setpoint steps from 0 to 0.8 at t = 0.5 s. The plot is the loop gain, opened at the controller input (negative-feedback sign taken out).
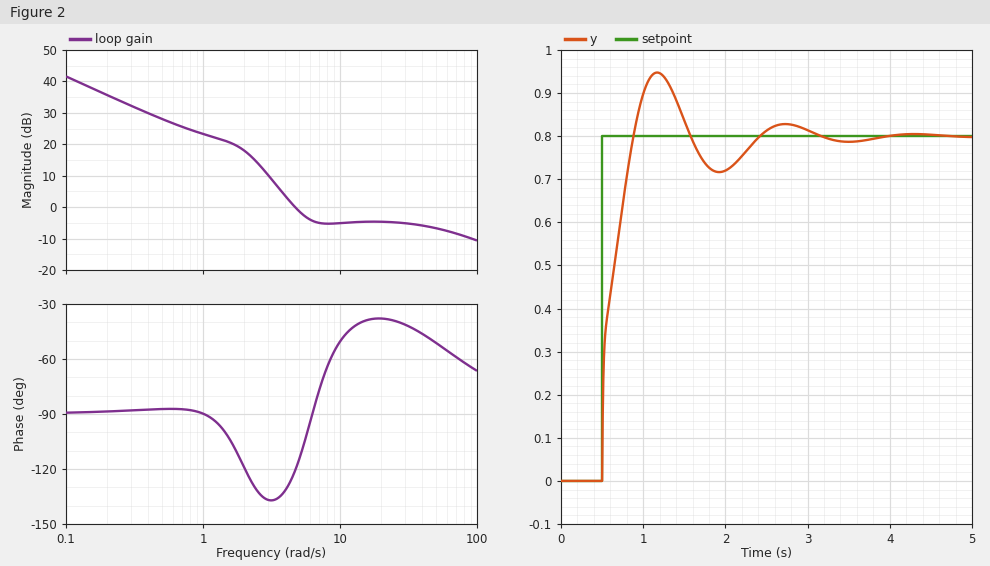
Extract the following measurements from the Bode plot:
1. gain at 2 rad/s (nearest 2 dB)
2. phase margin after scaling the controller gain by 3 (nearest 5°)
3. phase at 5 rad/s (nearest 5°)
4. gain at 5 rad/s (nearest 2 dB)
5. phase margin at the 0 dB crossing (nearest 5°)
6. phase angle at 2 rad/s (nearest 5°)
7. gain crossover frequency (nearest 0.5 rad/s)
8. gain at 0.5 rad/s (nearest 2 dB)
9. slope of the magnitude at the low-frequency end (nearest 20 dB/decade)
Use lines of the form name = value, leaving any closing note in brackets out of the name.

gain at 2 rad/s = 18 dB
phase margin after scaling the controller gain by 3 = 115°
phase at 5 rad/s = -115°
gain at 5 rad/s = -2 dB
phase margin at the 0 dB crossing = 60°
phase angle at 2 rad/s = -120°
gain crossover frequency = 4.5 rad/s
gain at 0.5 rad/s = 28 dB
slope of the magnitude at the low-frequency end = -20 dB/decade
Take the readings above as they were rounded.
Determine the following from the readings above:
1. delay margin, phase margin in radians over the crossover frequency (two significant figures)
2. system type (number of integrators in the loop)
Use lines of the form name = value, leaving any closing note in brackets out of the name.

delay margin, phase margin in radians over the crossover frequency = 0.23 s
system type = 1
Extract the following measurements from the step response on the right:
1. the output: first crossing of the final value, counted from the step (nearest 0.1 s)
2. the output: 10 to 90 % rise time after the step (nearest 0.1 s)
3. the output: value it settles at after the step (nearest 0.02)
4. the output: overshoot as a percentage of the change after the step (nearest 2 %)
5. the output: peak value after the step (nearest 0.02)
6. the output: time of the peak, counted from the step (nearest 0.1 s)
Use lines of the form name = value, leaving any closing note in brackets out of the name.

the output: first crossing of the final value, counted from the step = 0.4 s
the output: 10 to 90 % rise time after the step = 0.3 s
the output: value it settles at after the step = 0.80
the output: overshoot as a percentage of the change after the step = 18 %
the output: peak value after the step = 0.94
the output: time of the peak, counted from the step = 0.7 s
